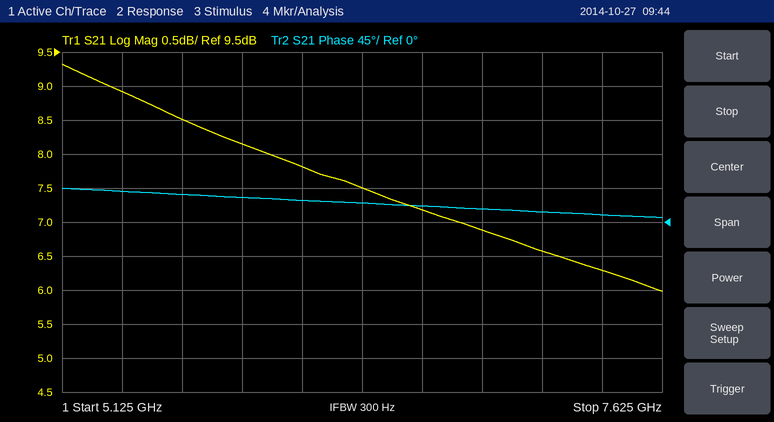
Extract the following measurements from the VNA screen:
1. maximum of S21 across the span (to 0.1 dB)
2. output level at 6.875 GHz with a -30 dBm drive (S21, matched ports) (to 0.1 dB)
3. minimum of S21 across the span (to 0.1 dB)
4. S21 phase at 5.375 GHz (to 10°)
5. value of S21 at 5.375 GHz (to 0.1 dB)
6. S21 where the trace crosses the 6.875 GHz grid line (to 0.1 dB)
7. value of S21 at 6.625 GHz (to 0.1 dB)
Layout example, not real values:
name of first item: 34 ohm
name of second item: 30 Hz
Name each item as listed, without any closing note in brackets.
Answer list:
maximum of S21 across the span: 9.3 dB
output level at 6.875 GHz with a -30 dBm drive (S21, matched ports): -23.1 dBm
minimum of S21 across the span: 6.0 dB
S21 phase at 5.375 GHz: 40°
value of S21 at 5.375 GHz: 8.9 dB
S21 where the trace crosses the 6.875 GHz grid line: 6.9 dB
value of S21 at 6.625 GHz: 7.2 dB
